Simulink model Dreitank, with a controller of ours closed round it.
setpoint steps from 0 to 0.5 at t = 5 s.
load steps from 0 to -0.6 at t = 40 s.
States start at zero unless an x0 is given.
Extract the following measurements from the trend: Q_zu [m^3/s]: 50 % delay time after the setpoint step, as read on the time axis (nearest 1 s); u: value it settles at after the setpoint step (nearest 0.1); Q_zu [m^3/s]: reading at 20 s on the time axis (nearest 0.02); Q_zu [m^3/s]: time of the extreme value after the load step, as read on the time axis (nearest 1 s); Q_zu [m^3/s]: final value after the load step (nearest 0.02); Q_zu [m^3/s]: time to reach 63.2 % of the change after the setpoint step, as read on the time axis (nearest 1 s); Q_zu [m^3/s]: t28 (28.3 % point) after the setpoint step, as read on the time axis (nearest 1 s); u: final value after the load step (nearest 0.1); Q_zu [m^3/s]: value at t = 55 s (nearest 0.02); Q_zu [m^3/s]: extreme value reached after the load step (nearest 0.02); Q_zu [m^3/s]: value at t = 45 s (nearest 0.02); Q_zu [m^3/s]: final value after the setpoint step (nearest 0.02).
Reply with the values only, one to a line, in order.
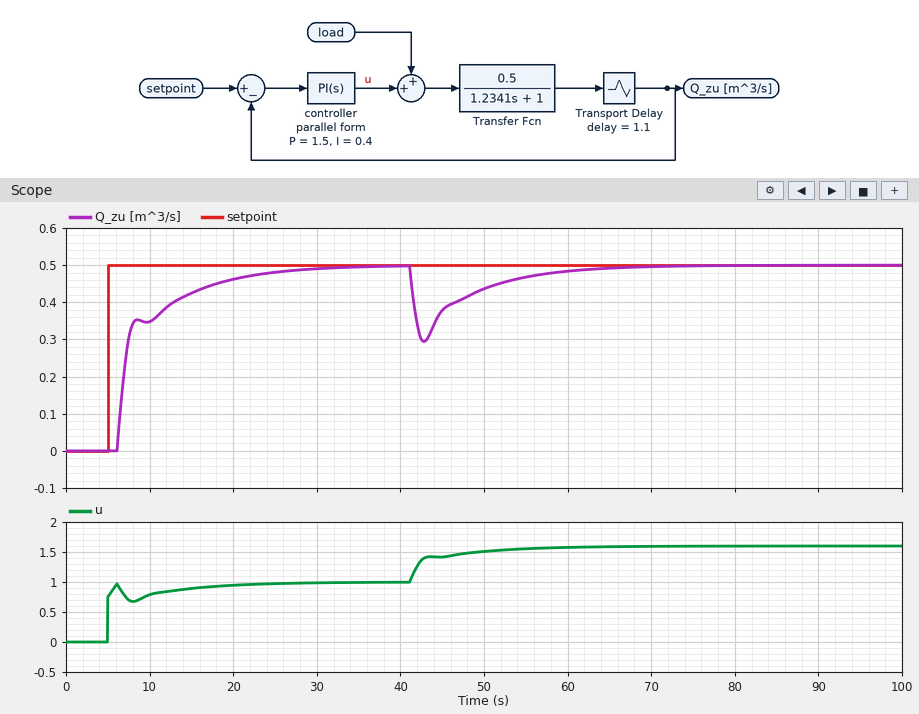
7 s
1.0
0.46
43 s
0.50
8 s
7 s
1.6
0.46
0.30
0.38
0.50
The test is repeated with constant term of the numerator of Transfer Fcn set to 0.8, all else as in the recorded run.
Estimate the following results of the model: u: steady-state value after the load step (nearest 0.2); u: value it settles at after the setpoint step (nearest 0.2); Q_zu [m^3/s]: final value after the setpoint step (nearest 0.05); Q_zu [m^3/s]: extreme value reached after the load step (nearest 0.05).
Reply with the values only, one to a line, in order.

1.2
0.6
0.50
0.20
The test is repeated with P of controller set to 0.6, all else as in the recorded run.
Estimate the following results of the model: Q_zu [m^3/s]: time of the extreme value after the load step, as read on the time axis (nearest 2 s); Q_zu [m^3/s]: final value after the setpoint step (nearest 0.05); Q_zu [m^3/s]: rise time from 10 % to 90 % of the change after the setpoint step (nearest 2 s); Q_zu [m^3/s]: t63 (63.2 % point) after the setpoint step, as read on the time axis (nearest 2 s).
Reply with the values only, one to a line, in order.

44 s
0.50
8 s
10 s
